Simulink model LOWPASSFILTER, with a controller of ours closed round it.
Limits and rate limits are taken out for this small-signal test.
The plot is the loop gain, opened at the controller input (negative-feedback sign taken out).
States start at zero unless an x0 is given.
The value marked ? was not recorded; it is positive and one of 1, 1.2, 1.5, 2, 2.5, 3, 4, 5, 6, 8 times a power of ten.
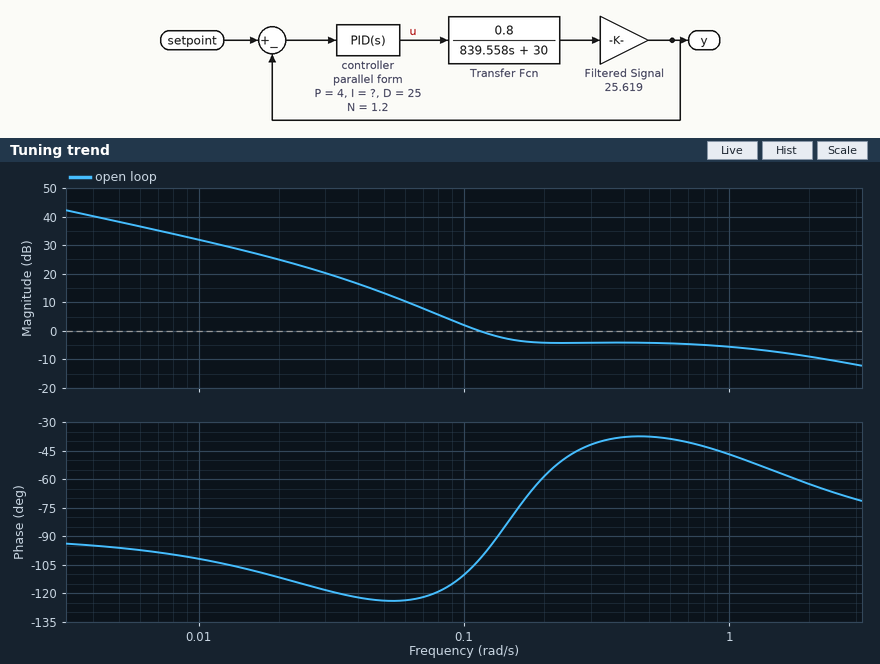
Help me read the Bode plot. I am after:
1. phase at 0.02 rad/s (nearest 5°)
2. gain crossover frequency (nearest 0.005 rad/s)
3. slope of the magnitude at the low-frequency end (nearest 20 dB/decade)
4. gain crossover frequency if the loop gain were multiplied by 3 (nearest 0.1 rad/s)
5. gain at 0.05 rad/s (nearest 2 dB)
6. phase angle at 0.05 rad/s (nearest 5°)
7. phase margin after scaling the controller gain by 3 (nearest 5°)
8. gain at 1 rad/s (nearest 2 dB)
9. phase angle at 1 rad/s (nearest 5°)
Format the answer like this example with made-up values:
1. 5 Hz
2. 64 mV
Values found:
1. -110°
2. 0.115 rad/s
3. -20 dB/decade
4. 2.2 rad/s
5. 14 dB
6. -125°
7. 115°
8. -6 dB
9. -45°
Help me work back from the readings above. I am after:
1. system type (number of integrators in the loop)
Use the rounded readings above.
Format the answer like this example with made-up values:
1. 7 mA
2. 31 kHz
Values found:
1. 1
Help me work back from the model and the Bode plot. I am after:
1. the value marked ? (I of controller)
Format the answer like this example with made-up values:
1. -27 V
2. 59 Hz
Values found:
1. 0.6
